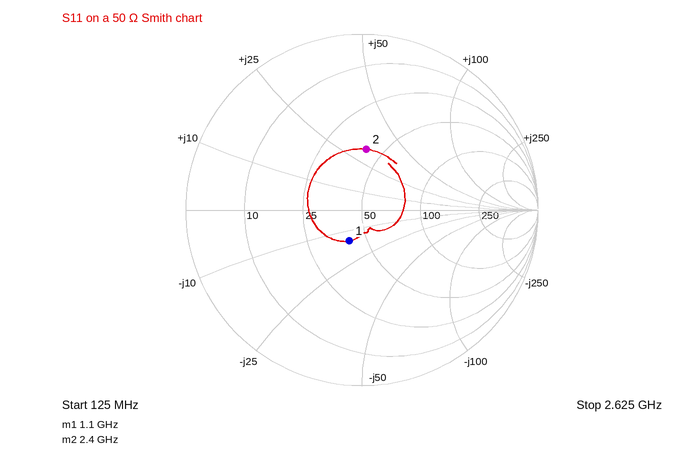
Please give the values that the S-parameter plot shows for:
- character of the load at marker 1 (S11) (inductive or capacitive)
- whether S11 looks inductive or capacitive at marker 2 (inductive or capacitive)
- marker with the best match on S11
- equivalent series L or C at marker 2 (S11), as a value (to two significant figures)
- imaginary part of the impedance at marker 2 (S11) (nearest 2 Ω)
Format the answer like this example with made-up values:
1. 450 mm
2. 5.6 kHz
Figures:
1. capacitive
2. inductive
3. marker 1
4. 2.1 nH
5. +32 Ω
